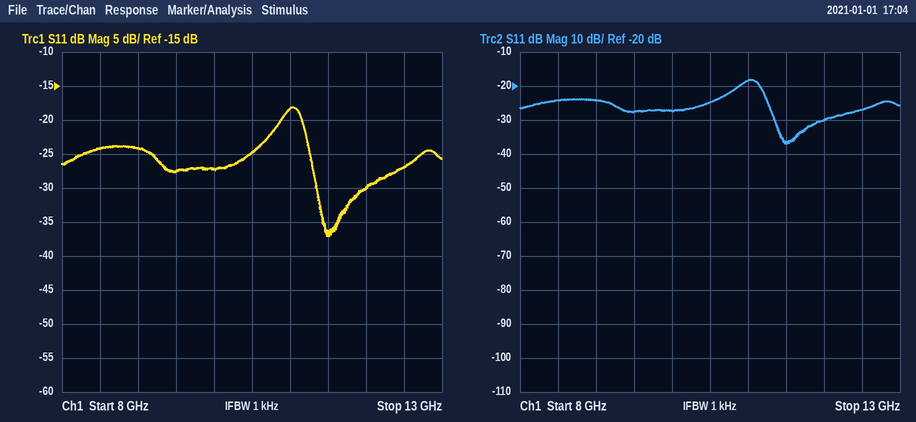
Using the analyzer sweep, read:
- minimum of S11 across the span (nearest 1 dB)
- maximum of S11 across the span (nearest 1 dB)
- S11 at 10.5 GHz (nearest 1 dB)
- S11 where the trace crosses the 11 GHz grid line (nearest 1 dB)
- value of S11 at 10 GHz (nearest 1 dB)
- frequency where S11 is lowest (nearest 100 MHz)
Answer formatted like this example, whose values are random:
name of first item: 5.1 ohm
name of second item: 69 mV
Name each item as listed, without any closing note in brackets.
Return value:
minimum of S11 across the span: -37 dB
maximum of S11 across the span: -18 dB
S11 at 10.5 GHz: -25 dB
S11 where the trace crosses the 11 GHz grid line: -18 dB
value of S11 at 10 GHz: -27 dB
frequency where S11 is lowest: 11.5 GHz
